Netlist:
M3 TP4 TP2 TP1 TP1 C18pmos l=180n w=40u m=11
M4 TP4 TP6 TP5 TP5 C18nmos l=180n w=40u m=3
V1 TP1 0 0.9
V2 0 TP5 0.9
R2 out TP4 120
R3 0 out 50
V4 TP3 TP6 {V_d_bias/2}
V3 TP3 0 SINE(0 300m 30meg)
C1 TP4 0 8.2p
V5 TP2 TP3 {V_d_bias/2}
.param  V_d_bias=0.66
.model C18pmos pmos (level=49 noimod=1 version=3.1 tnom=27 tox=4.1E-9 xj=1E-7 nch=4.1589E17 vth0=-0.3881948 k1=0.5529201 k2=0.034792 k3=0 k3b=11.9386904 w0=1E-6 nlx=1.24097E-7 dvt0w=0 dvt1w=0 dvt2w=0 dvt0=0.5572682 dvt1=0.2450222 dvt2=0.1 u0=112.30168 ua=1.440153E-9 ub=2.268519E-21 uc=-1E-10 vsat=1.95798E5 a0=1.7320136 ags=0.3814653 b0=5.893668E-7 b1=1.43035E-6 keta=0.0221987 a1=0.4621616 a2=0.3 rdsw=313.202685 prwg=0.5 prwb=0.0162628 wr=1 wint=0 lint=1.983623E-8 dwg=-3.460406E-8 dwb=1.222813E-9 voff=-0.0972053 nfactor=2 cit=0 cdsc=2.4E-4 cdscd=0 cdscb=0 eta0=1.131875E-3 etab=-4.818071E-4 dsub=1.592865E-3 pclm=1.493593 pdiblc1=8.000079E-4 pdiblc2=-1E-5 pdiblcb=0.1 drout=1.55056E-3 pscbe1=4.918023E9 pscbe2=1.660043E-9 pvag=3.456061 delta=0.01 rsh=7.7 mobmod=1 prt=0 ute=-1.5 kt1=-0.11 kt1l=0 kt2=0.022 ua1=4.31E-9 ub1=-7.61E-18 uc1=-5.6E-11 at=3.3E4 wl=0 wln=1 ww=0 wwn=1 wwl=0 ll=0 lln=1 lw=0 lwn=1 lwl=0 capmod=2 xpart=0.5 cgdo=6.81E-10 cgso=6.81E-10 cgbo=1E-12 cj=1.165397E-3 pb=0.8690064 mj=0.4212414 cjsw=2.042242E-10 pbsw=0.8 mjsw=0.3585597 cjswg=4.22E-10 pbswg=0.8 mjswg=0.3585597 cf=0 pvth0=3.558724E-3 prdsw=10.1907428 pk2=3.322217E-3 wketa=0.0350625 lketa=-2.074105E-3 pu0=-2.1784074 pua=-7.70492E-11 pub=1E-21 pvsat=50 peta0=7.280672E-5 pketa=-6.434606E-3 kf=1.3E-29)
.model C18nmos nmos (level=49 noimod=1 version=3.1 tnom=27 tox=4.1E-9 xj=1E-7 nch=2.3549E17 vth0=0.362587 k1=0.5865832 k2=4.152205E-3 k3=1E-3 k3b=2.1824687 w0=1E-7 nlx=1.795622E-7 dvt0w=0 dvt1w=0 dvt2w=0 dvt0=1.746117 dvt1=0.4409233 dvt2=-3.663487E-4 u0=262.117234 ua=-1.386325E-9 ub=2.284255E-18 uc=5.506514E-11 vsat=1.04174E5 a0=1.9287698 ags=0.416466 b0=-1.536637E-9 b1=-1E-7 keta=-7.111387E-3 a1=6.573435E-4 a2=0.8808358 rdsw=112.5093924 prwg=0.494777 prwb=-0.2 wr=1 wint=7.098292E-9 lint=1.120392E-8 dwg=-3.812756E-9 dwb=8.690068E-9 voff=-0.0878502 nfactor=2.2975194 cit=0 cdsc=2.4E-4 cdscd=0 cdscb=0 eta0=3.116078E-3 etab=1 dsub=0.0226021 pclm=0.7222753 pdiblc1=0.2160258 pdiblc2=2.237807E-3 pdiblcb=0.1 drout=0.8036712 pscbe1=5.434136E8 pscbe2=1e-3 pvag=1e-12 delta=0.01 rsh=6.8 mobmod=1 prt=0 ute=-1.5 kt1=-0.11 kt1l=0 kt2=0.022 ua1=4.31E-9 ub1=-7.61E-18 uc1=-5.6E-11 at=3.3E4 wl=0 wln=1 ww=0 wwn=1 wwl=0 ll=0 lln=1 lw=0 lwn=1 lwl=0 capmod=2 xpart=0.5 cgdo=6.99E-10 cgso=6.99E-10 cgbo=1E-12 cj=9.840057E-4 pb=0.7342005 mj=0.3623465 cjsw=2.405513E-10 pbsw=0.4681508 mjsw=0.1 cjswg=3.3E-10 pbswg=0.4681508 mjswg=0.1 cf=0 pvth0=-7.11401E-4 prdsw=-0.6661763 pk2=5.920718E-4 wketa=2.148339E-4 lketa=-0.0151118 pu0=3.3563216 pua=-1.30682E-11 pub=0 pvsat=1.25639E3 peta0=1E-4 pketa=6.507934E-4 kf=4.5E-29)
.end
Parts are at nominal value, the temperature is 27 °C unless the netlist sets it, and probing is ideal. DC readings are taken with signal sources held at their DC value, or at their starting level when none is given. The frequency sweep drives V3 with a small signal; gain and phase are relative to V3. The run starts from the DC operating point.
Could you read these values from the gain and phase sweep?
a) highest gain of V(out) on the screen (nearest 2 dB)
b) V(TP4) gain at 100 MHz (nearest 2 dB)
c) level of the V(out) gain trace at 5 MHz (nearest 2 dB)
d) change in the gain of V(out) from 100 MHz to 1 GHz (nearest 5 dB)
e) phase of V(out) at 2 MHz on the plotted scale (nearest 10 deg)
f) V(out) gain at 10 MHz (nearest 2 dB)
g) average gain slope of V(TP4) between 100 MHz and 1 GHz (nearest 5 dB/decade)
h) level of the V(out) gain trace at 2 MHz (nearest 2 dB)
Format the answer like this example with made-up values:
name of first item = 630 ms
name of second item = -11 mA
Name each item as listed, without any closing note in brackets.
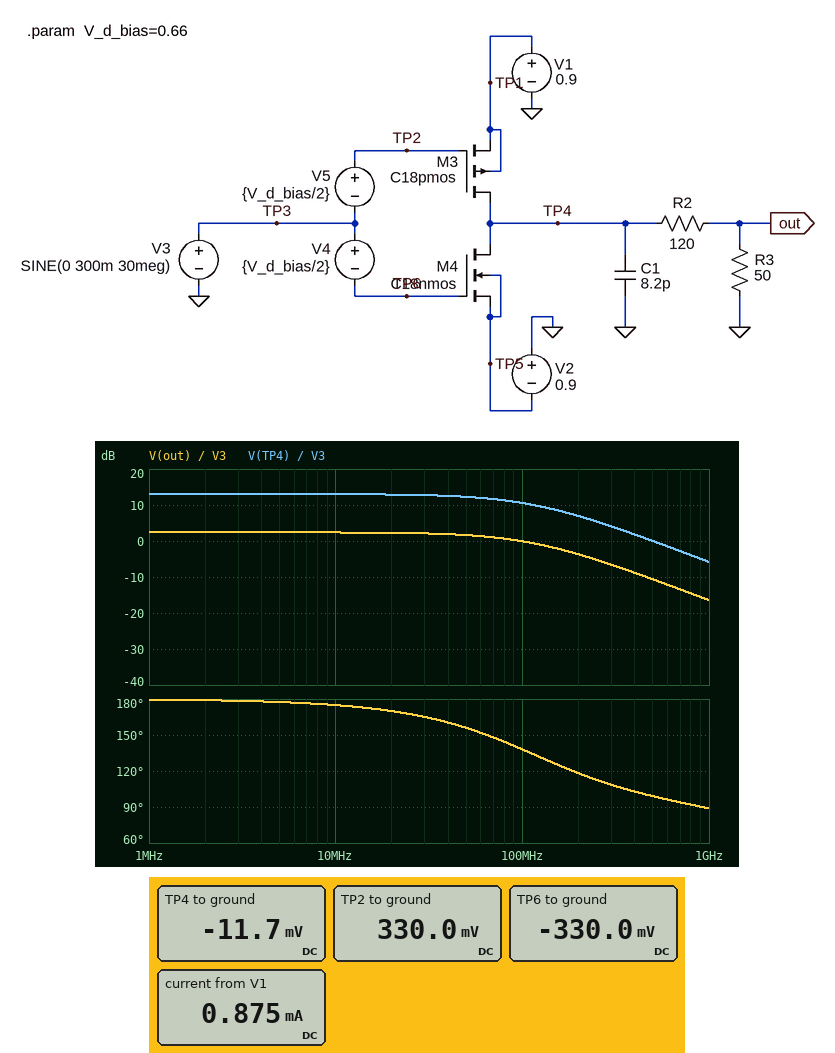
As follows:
highest gain of V(out) on the screen = 2 dB
V(TP4) gain at 100 MHz = 10 dB
level of the V(out) gain trace at 5 MHz = 2 dB
change in the gain of V(out) from 100 MHz to 1 GHz = -15 dB
phase of V(out) at 2 MHz on the plotted scale = 180 deg
V(out) gain at 10 MHz = 2 dB
average gain slope of V(TP4) between 100 MHz and 1 GHz = -15 dB/decade
level of the V(out) gain trace at 2 MHz = 2 dB
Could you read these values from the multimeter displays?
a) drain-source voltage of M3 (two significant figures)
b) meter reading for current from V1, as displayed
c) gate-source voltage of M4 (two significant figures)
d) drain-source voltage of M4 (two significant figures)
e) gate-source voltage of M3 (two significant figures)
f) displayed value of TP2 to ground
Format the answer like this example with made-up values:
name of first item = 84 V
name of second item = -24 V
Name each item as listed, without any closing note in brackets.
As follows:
drain-source voltage of M3 = -910 mV
meter reading for current from V1, as displayed = 0.875 mA
gate-source voltage of M4 = 570 mV
drain-source voltage of M4 = 890 mV
gate-source voltage of M3 = -570 mV
displayed value of TP2 to ground = 330.0 mV
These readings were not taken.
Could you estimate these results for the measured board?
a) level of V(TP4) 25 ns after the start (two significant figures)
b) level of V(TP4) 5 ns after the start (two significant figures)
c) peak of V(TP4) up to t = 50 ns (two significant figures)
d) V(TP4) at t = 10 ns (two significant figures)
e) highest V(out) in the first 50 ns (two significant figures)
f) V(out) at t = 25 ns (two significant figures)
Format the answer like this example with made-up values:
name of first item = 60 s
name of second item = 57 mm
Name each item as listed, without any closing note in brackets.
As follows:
level of V(TP4) 25 ns after the start = 810 mV
level of V(TP4) 5 ns after the start = -770 mV
peak of V(TP4) up to t = 50 ns = 810 mV
V(TP4) at t = 10 ns = -790 mV
highest V(out) in the first 50 ns = 240 mV
V(out) at t = 25 ns = 240 mV
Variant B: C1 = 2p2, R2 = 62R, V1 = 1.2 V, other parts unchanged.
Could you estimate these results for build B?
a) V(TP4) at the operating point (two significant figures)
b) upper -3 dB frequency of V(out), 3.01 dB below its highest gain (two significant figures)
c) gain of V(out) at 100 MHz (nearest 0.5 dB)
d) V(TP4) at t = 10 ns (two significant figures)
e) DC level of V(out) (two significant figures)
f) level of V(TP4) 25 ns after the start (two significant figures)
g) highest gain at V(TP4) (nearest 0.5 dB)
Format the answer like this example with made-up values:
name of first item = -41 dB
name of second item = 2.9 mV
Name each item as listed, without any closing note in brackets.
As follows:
V(TP4) at the operating point = 950 mV
upper -3 dB frequency of V(out), 3.01 dB below its highest gain = 1.6 GHz
gain of V(out) at 100 MHz = -1.0 dB
V(TP4) at t = 10 ns = -690 mV
DC level of V(out) = 420 mV
level of V(TP4) 25 ns after the start = 1.1 V
highest gain at V(TP4) = 6.0 dB
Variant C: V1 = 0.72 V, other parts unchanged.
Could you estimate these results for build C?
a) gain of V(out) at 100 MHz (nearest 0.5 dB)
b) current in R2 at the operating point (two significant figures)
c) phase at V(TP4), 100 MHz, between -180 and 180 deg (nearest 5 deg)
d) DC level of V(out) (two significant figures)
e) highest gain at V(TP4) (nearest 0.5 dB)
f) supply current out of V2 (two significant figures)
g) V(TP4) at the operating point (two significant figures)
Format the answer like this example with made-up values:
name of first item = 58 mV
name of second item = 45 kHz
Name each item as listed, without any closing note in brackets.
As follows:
gain of V(out) at 100 MHz = -6.0 dB
current in R2 at the operating point = 890 µA
phase at V(TP4), 100 MHz, between -180 and 180 deg = 135 deg
DC level of V(out) = -44 mV
highest gain at V(TP4) = 7.0 dB
supply current out of V2 = 910 µA
V(TP4) at the operating point = -150 mV
